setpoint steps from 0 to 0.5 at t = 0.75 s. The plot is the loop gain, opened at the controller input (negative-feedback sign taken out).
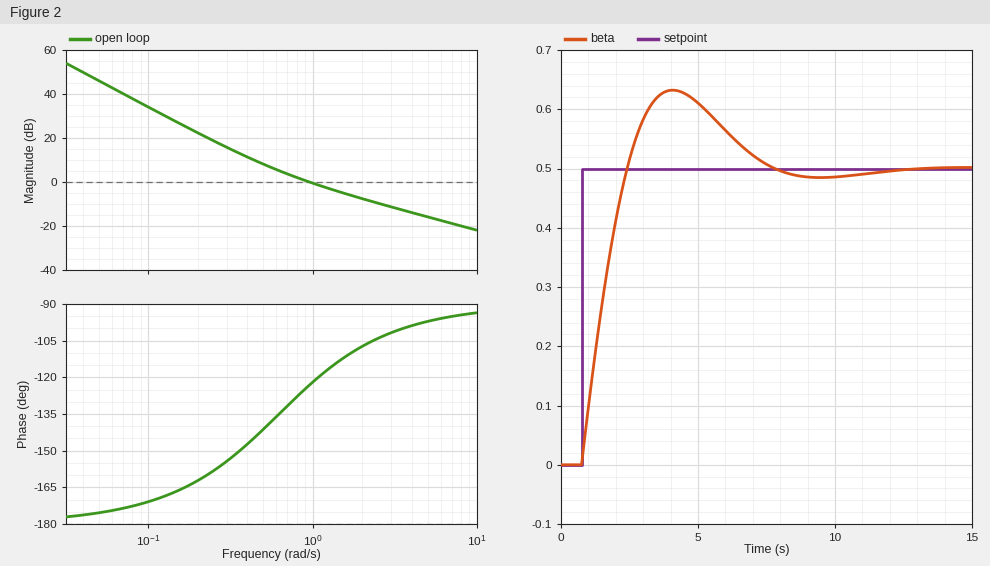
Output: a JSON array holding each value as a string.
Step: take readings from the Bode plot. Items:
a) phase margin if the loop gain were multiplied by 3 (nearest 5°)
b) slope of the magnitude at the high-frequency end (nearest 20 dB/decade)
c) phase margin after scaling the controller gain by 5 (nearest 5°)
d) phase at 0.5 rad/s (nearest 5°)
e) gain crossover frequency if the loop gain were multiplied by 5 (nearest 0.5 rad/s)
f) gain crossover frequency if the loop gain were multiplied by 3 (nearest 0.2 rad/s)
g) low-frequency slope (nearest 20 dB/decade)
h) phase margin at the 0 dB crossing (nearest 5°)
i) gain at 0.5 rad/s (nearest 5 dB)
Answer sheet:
["75°", "-20 dB/decade", "80°", "-140°", "4.0 rad/s", "2.4 rad/s", "-40 dB/decade", "55°", "10 dB"]
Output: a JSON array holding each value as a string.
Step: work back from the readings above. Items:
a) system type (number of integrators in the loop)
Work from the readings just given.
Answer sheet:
["2"]
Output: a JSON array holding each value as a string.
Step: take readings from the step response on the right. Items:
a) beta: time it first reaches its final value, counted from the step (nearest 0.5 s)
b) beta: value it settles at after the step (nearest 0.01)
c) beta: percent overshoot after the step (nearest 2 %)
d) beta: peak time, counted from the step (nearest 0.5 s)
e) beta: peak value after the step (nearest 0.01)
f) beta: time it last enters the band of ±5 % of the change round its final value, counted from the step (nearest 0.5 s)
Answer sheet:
["1.5 s", "0.50", "26 %", "3.5 s", "0.63", "6.0 s"]
